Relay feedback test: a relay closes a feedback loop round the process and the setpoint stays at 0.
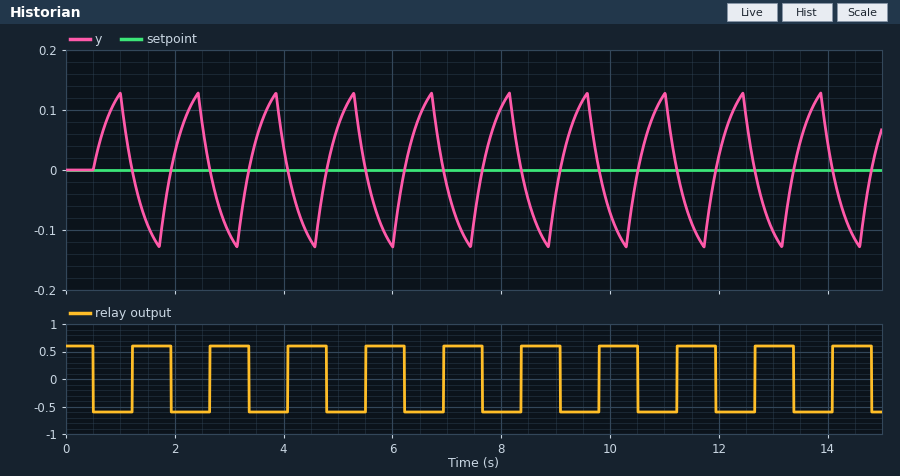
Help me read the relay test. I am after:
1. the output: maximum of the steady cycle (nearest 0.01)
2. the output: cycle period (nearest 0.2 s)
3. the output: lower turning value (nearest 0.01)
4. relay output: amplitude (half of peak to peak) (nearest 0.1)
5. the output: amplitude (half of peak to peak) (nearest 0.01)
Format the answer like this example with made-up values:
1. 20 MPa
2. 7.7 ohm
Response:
1. 0.13
2. 1.4 s
3. -0.13
4. 0.6
5. 0.13
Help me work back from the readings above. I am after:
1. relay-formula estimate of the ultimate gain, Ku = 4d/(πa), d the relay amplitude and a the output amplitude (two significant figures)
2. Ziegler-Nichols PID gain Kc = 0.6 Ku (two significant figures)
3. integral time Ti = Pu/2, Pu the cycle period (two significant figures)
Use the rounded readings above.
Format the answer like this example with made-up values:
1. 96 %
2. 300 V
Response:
1. 5.9
2. 3.5
3. 0.70 s
